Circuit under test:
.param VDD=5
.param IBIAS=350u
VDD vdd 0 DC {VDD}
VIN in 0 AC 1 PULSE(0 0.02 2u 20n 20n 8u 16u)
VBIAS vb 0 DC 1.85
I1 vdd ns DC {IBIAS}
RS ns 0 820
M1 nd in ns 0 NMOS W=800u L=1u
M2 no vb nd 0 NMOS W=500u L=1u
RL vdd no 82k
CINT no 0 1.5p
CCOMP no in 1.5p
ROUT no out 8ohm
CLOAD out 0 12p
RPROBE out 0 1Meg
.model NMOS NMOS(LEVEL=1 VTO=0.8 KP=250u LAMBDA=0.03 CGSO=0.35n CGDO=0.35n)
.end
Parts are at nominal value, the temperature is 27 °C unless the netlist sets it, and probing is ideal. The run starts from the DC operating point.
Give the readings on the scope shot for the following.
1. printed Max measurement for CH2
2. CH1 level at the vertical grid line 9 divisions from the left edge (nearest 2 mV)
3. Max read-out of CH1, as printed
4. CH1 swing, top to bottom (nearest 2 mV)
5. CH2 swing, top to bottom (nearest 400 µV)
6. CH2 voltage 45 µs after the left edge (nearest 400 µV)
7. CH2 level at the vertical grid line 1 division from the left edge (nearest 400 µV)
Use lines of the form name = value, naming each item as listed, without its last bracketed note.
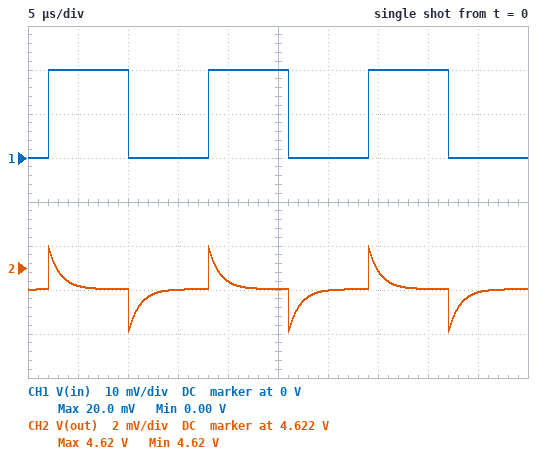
printed Max measurement for CH2 = 4.62 V
CH1 level at the vertical grid line 9 divisions from the left edge = 0 V
Max read-out of CH1, as printed = 20.0 mV
CH1 swing, top to bottom = 20 mV
CH2 swing, top to bottom = 4.0 mV
CH2 voltage 45 µs after the left edge = 4.6208 V
CH2 level at the vertical grid line 1 division from the left edge = 4.6212 V
